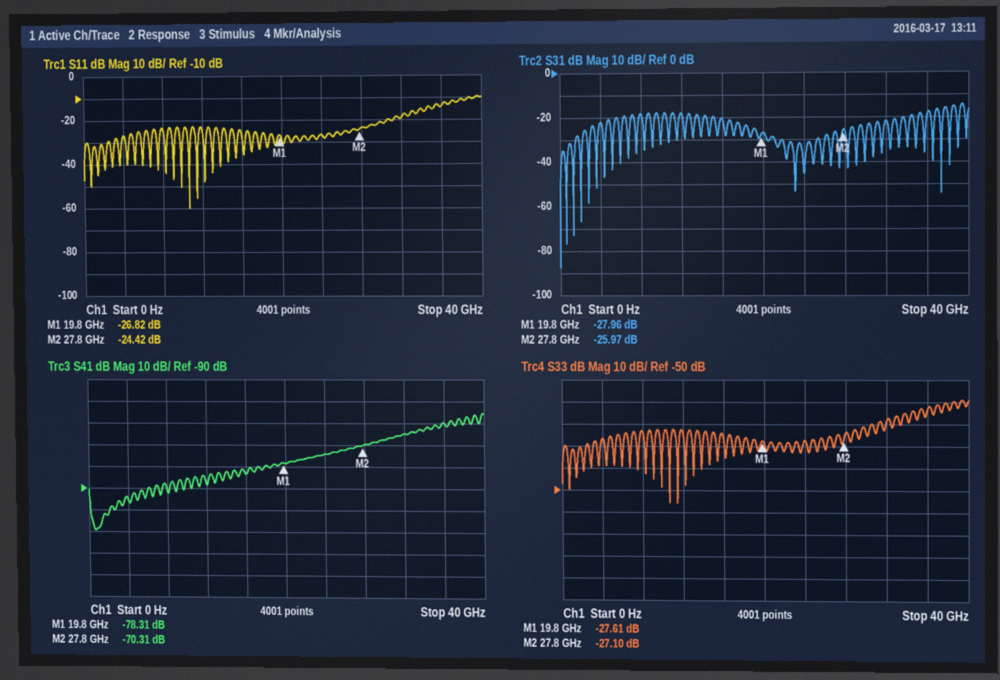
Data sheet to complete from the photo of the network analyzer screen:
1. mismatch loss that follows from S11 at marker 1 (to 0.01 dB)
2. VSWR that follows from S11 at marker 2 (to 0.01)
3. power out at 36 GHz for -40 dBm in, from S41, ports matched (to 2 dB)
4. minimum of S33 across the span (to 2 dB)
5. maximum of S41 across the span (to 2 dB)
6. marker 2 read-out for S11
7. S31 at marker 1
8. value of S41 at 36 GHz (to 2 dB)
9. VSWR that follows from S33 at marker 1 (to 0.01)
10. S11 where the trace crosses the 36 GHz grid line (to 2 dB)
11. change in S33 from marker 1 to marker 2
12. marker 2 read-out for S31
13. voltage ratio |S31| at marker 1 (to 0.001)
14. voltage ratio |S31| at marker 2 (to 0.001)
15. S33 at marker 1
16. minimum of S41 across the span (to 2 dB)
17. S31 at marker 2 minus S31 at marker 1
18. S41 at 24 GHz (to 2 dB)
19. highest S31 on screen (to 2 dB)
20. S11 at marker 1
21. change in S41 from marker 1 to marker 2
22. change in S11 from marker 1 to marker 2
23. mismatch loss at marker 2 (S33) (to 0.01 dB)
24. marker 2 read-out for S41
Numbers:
0.01 dB
1.13
-100 dBm
-56 dB
-56 dB
-24.42 dB
-27.96 dB
-60 dB
1.09
-14 dB
0.51 dB
-25.97 dB
0.040
0.050
-27.61 dB
-110 dB
1.99 dB
-74 dB
-14 dB
-26.82 dB
8.00 dB
2.40 dB
0.01 dB
-70.31 dB
